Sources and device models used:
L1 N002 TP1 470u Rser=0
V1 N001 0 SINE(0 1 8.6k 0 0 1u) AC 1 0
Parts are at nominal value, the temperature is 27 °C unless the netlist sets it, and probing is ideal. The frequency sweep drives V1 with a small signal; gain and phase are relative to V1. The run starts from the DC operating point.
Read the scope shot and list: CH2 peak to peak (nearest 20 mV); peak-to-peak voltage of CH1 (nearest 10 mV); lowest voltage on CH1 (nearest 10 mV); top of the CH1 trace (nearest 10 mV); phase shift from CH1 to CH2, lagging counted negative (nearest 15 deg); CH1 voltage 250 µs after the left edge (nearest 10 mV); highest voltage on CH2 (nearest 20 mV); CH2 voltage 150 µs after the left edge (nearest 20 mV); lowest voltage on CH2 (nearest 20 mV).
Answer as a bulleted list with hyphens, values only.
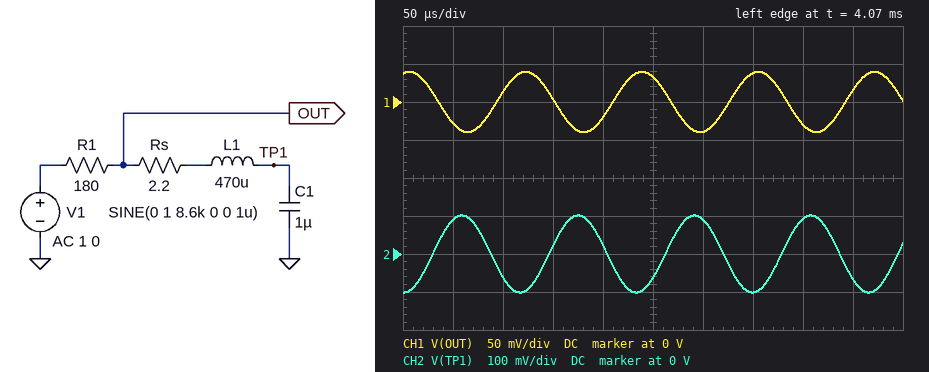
- 200 mV
- 80 mV
- -40 mV
- 40 mV
- -165 deg
- 30 mV
- 100 mV
- 20 mV
- -100 mV
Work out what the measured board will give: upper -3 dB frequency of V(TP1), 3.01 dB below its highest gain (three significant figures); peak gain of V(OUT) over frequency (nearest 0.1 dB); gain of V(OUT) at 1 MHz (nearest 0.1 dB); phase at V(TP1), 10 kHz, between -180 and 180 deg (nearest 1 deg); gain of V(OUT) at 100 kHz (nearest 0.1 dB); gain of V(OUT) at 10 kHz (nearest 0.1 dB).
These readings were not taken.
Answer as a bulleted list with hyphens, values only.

- 886 Hz
- 0 dB
- 0 dB
- -94 deg
- -1.4 dB
- -22.4 dB
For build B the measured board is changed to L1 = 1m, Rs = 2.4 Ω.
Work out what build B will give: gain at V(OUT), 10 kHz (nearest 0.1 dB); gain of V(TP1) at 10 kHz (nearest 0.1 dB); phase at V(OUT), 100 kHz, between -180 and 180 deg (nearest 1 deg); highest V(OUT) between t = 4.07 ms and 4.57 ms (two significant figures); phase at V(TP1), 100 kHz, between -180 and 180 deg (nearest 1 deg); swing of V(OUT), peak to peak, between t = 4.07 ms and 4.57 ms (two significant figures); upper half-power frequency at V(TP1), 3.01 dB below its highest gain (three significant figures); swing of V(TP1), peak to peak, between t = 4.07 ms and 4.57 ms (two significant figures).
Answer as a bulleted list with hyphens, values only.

- -12.1 dB
- -21.5 dB
- 16 deg
- 190 mV
- -164 deg
- 380 mV
- 900 Hz
- 200 mV
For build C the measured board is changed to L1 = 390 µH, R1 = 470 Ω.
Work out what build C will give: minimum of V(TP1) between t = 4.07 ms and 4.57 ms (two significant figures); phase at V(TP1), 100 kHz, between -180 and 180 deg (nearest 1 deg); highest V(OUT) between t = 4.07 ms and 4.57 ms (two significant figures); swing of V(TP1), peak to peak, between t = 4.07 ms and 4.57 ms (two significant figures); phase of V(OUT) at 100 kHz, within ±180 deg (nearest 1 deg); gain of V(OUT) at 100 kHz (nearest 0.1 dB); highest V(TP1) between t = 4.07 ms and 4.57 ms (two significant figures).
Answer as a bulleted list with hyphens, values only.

- -39 mV
- -117 deg
- 7.2 mV
- 78 mV
- 62 deg
- -6.8 dB
- 39 mV
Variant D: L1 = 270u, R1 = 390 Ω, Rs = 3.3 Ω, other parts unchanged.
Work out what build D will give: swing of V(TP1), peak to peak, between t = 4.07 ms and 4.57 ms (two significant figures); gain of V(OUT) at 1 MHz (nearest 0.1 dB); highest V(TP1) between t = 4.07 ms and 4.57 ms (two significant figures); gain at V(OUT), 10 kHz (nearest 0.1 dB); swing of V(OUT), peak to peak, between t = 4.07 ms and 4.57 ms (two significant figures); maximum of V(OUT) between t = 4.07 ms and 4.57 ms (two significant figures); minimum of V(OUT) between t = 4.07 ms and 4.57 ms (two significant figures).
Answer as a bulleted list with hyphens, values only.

- 94 mV
- -0.2 dB
- 47 mV
- -41.1 dB
- 26 mV
- 13 mV
- -13 mV
